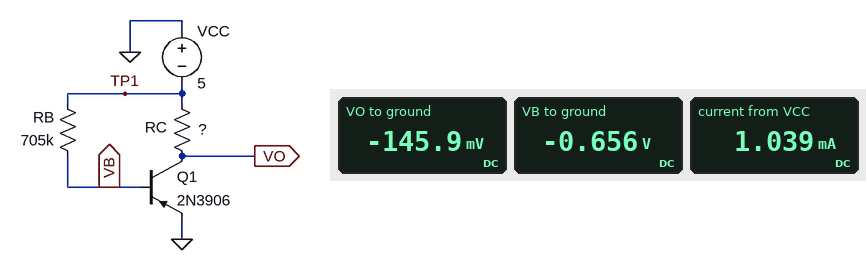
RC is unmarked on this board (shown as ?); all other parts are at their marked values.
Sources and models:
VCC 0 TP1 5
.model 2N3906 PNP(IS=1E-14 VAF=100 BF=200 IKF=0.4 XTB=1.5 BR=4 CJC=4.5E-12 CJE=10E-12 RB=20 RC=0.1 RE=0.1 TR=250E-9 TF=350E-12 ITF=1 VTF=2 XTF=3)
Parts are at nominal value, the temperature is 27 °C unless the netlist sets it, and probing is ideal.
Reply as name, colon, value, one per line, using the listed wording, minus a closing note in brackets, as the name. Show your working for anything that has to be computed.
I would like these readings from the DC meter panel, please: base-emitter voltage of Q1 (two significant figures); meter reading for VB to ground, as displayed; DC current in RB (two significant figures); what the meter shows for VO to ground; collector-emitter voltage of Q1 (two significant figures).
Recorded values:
base-emitter voltage of Q1: -656 mV = -660 mV
meter reading for VB to ground, as displayed: -0.656 V
DC current in RB: (-656 mV - (-5 V)) / 705 kΩ = 6.2 µA
what the meter shows for VO to ground: -145.9 mV
collector-emitter voltage of Q1: -145.9 mV = -150 mV
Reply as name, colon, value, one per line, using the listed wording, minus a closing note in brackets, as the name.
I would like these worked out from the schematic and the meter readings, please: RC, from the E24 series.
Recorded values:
RC, from the E24 series: 4.7 kΩ
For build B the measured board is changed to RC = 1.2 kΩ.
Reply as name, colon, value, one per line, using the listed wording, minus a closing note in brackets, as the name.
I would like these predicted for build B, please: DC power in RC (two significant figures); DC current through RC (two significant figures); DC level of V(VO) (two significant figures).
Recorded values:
DC power in RC: 1.9 mW
DC current through RC: 1.3 mA
DC level of V(VO): -3.5 V
